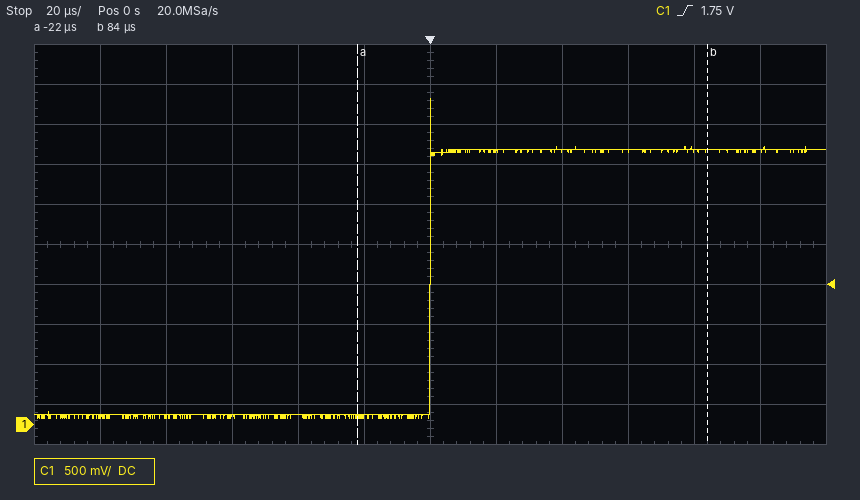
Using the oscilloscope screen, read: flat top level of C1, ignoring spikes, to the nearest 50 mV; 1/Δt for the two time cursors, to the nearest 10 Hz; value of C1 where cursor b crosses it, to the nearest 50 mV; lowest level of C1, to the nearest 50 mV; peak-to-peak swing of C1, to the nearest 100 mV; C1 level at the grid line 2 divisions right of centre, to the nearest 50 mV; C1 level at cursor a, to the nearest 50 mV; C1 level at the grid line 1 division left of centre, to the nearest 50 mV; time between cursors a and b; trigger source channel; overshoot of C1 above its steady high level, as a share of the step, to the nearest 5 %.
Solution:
3.45 V
9.43 kHz
3.40 V
100 mV
4.00 V
3.40 V
100 mV
100 mV
106 µs
C1
20 %
